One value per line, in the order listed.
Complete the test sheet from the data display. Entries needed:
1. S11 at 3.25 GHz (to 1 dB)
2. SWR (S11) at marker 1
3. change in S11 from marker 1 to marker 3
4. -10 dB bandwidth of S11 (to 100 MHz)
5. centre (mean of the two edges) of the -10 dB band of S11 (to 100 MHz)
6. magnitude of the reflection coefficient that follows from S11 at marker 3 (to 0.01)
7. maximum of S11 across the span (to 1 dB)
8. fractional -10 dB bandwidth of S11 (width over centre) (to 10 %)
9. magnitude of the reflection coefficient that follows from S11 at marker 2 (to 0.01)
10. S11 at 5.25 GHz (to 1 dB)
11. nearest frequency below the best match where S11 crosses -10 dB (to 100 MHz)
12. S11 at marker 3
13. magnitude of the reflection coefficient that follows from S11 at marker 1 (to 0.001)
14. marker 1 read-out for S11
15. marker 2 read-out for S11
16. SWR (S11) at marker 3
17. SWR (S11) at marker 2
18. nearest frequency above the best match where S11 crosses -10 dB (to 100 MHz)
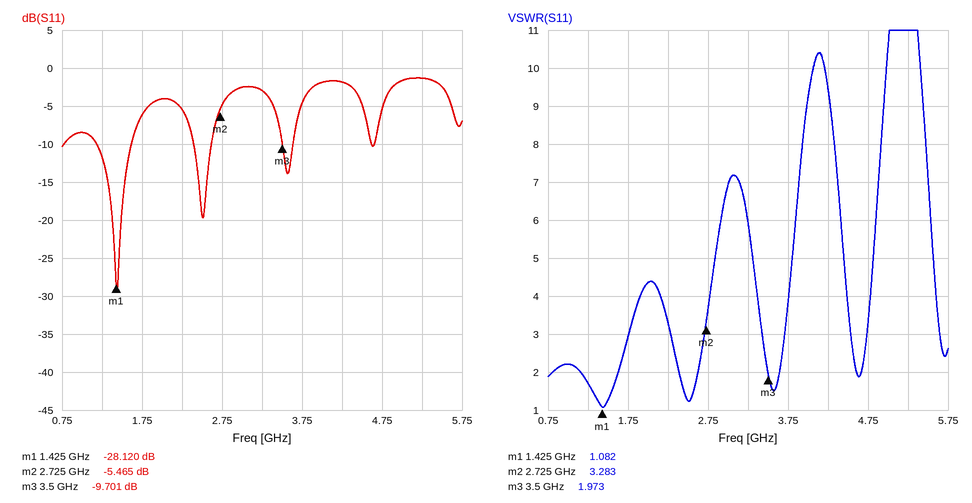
-3 dB
1.082
18.419 dB
400 MHz
1.4 GHz
0.33
-1 dB
30 %
0.53
-1 dB
1.2 GHz
-9.701 dB
0.039
-28.120 dB
-5.465 dB
1.973
3.283
1.6 GHz
